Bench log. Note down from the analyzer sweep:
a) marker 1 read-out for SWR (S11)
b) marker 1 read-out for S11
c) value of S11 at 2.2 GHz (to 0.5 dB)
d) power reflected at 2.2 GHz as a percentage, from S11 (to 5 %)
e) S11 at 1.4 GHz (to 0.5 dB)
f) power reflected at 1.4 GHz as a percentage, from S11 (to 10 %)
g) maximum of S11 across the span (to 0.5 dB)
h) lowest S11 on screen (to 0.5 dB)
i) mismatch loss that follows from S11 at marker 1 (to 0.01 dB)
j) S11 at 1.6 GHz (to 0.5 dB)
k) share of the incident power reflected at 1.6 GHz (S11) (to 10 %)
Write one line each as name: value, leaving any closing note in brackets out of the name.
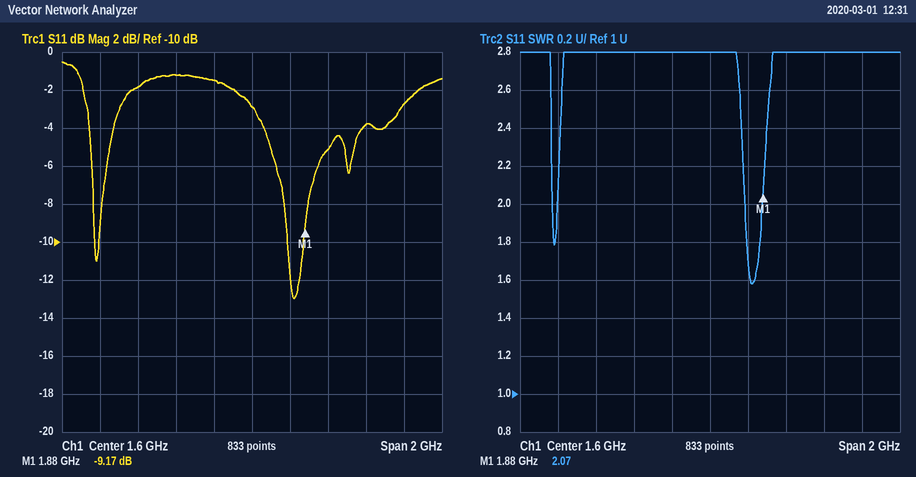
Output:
marker 1 read-out for SWR: 2.07
marker 1 read-out for S11: -9.17 dB
value of S11 at 2.2 GHz: -4.0 dB
power reflected at 2.2 GHz as a percentage, from S11: 40 %
S11 at 1.4 GHz: -1.5 dB
power reflected at 1.4 GHz as a percentage, from S11: 70 %
maximum of S11 across the span: -0.5 dB
lowest S11 on screen: -13.0 dB
mismatch loss that follows from S11 at marker 1: 0.56 dB
S11 at 1.6 GHz: -3.0 dB
share of the incident power reflected at 1.6 GHz (S11): 50 %
